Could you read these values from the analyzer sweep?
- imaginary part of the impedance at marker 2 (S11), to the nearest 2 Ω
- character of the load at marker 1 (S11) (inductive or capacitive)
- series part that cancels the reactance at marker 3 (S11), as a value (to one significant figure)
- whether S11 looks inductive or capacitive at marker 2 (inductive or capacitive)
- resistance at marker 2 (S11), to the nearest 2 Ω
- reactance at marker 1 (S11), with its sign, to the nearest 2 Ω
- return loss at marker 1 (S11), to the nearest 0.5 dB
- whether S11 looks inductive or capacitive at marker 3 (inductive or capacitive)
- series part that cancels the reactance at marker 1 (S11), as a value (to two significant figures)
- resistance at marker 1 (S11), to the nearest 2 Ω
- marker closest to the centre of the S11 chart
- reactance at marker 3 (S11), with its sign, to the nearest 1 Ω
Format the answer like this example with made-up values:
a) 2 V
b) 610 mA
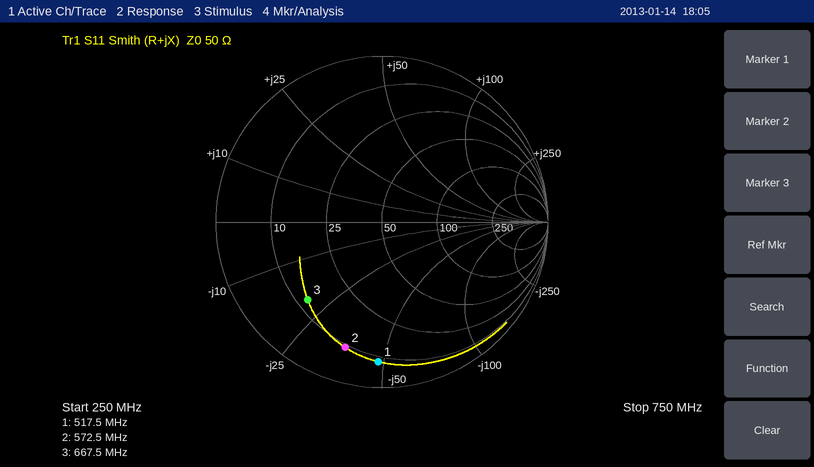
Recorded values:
a) -36 Ω
b) capacitive
c) 5 nH
d) capacitive
e) 10 Ω
f) -48 Ω
g) 1.5 dB
h) capacitive
i) 15 nH
j) 8 Ω
k) marker 3
l) -20 Ω
